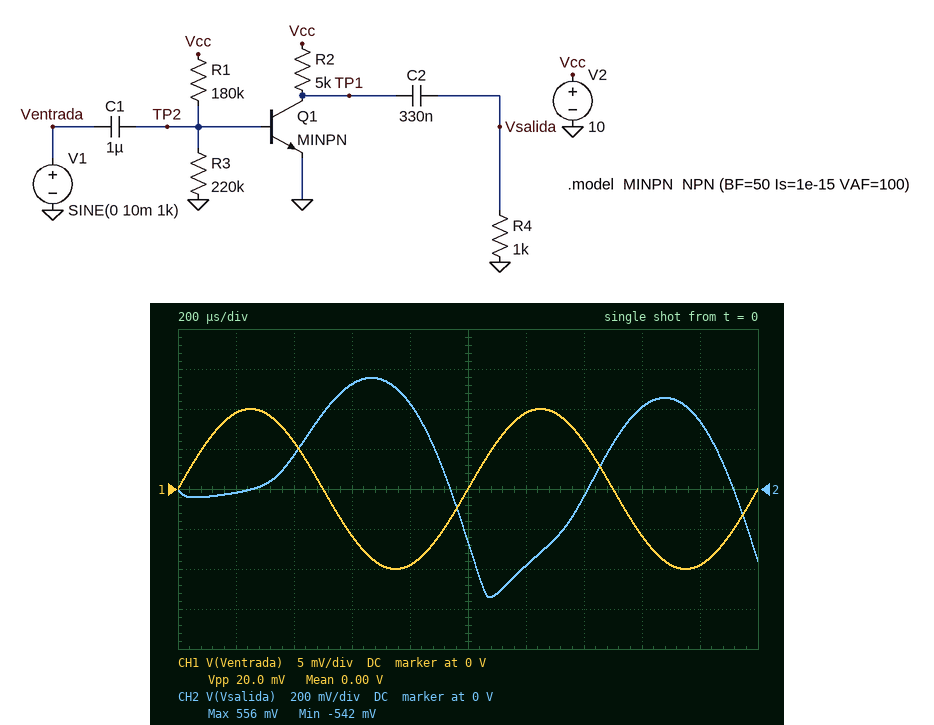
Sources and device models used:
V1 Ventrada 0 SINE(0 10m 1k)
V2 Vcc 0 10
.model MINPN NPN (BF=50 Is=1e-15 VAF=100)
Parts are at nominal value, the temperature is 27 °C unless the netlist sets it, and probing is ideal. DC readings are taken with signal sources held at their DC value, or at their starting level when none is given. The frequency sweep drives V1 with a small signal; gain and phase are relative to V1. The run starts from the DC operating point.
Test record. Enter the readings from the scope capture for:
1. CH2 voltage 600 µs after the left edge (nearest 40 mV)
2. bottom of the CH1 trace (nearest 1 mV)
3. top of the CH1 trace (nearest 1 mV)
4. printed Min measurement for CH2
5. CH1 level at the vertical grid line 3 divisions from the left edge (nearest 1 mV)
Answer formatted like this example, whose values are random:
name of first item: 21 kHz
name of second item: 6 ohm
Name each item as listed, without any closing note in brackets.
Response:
CH2 voltage 600 µs after the left edge: 520 mV
bottom of the CH1 trace: -10 mV
top of the CH1 trace: 10 mV
printed Min measurement for CH2: -542 mV
CH1 level at the vertical grid line 3 divisions from the left edge: -6 mV
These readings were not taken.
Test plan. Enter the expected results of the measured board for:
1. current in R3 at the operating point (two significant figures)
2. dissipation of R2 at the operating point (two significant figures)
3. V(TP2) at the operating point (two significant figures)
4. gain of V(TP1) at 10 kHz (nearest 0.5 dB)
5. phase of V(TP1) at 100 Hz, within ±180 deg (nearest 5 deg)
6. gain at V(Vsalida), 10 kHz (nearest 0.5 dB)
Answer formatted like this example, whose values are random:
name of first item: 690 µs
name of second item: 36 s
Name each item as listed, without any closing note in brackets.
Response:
current in R3 at the operating point: 3.3 µA
dissipation of R2 at the operating point: 19 mW
V(TP2) at the operating point: 730 mV
gain of V(TP1) at 10 kHz: 32.0 dB
phase of V(TP1) at 100 Hz, within ±180 deg: -90 deg
gain at V(Vsalida), 10 kHz: 32.0 dB
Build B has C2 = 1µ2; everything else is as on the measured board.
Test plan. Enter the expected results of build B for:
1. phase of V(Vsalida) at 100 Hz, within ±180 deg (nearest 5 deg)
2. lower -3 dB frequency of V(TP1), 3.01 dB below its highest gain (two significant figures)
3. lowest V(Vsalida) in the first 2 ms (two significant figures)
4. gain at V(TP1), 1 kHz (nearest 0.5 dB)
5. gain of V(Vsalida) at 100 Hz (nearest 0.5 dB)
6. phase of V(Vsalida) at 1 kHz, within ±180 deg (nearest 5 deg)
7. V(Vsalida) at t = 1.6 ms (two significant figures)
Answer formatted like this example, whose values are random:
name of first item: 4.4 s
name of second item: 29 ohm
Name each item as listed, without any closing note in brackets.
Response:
phase of V(Vsalida) at 100 Hz, within ±180 deg: -40 deg
lower -3 dB frequency of V(TP1), 3.01 dB below its highest gain: 2.3 kHz
lowest V(Vsalida) in the first 2 ms: -260 mV
gain at V(TP1), 1 kHz: 24.5 dB
gain of V(Vsalida) at 100 Hz: 1.0 dB
phase of V(Vsalida) at 1 kHz, within ±180 deg: -105 deg
V(Vsalida) at t = 1.6 ms: 480 mV
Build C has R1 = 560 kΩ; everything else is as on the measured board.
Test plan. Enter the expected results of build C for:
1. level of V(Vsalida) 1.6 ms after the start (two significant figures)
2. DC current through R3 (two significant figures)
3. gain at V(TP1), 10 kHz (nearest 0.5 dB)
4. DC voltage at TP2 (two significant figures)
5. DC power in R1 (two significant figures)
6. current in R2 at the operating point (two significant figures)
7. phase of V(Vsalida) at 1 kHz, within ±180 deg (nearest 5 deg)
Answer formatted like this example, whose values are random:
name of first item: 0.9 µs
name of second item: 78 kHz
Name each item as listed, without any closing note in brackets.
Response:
level of V(Vsalida) 1.6 ms after the start: 170 mV
DC current through R3: 3.2 µA
gain at V(TP1), 10 kHz: 27.0 dB
DC voltage at TP2: 700 mV
DC power in R1: 150 µW
current in R2 at the operating point: 710 µA
phase of V(Vsalida) at 1 kHz, within ±180 deg: -170 deg
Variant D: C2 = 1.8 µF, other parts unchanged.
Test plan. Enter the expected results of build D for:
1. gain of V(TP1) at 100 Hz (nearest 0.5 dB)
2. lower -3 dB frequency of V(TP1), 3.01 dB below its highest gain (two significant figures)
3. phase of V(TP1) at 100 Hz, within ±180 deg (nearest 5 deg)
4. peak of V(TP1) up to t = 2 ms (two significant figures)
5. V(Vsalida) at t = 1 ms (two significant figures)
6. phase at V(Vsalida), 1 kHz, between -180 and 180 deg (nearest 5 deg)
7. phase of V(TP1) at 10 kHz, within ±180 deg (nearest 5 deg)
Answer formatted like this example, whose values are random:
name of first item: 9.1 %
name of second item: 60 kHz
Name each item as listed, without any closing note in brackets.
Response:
gain of V(TP1) at 100 Hz: 5.0 dB
lower -3 dB frequency of V(TP1), 3.01 dB below its highest gain: 2.3 kHz
phase of V(TP1) at 100 Hz, within ±180 deg: -95 deg
peak of V(TP1) up to t = 2 ms: 860 mV
V(Vsalida) at t = 1 ms: -140 mV
phase at V(Vsalida), 1 kHz, between -180 and 180 deg: -110 deg
phase of V(TP1) at 10 kHz, within ±180 deg: -165 deg
